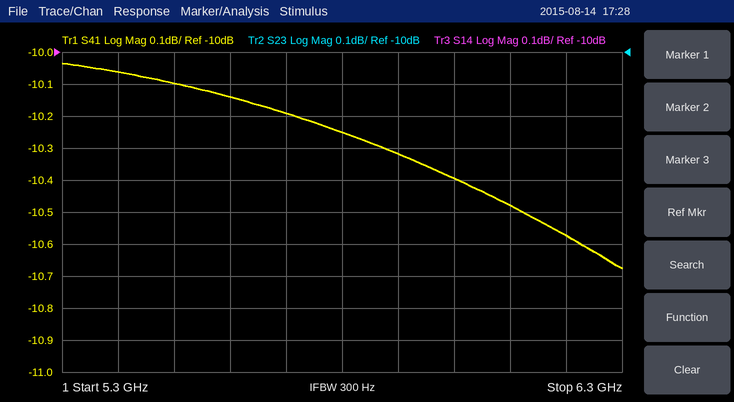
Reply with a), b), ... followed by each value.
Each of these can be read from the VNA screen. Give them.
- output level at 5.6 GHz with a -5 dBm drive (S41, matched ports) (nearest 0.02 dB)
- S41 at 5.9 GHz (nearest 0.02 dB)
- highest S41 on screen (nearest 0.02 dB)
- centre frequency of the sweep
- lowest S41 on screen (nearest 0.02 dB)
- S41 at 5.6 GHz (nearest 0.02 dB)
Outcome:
a) -15.14 dBm
b) -10.32 dB
c) -10.04 dB
d) 5.8 GHz
e) -10.68 dB
f) -10.14 dB
